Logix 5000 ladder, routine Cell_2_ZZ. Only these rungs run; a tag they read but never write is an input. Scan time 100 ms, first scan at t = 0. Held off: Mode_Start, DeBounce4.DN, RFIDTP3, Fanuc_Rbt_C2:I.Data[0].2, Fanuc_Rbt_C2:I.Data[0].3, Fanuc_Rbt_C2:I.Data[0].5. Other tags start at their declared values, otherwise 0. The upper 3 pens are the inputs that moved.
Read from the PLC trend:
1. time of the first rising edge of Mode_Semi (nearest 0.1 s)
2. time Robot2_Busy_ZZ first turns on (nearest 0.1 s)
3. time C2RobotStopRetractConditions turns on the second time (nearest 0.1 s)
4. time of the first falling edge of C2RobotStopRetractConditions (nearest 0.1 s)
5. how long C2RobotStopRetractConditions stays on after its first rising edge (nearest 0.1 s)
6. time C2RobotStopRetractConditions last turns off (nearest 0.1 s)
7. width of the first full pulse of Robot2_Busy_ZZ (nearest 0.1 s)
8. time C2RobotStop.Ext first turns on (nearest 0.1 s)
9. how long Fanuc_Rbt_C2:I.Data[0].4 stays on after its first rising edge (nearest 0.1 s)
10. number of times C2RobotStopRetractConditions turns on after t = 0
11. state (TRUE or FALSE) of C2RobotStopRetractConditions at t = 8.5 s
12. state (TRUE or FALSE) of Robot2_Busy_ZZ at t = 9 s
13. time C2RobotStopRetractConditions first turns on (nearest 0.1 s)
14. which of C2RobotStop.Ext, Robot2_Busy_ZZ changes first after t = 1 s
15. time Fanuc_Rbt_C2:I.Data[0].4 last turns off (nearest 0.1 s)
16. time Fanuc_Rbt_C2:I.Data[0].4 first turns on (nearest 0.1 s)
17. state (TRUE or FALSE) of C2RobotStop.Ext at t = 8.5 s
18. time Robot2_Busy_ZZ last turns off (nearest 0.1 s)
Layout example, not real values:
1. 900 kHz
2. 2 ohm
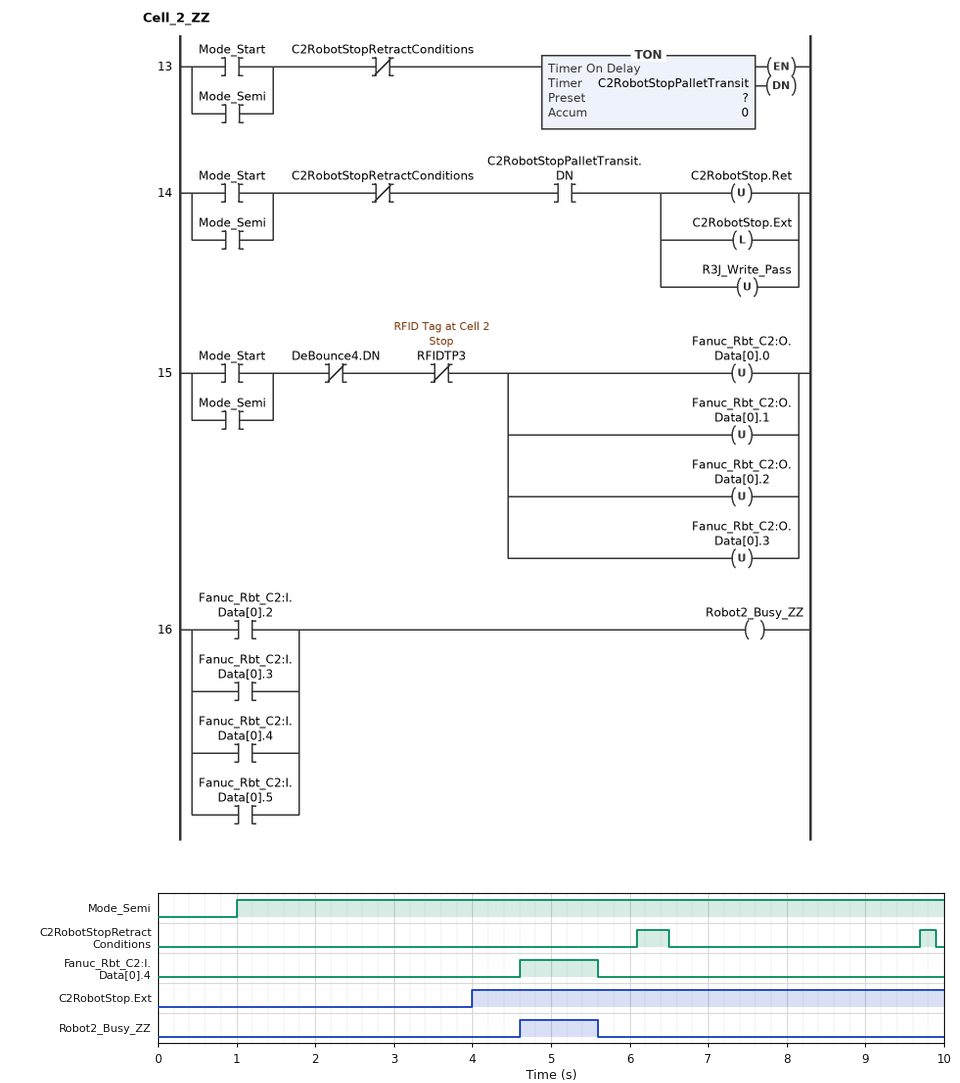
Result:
1. 1.0 s
2. 4.6 s
3. 9.7 s
4. 6.5 s
5. 0.4 s
6. 9.9 s
7. 1.0 s
8. 4.0 s
9. 1.0 s
10. 2
11. FALSE
12. FALSE
13. 6.1 s
14. C2RobotStop.Ext
15. 5.6 s
16. 4.6 s
17. TRUE
18. 5.6 s
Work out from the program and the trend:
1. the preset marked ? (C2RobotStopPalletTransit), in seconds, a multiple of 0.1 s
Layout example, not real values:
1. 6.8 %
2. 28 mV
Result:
1. 3.0 s
